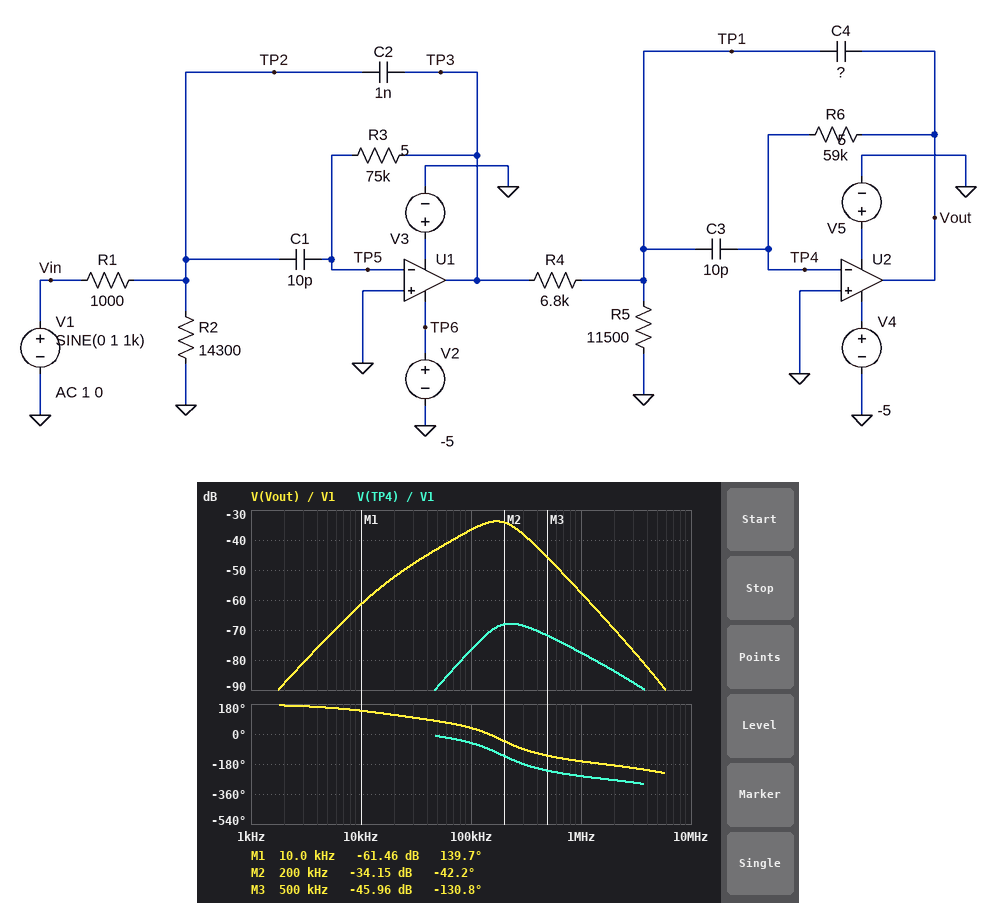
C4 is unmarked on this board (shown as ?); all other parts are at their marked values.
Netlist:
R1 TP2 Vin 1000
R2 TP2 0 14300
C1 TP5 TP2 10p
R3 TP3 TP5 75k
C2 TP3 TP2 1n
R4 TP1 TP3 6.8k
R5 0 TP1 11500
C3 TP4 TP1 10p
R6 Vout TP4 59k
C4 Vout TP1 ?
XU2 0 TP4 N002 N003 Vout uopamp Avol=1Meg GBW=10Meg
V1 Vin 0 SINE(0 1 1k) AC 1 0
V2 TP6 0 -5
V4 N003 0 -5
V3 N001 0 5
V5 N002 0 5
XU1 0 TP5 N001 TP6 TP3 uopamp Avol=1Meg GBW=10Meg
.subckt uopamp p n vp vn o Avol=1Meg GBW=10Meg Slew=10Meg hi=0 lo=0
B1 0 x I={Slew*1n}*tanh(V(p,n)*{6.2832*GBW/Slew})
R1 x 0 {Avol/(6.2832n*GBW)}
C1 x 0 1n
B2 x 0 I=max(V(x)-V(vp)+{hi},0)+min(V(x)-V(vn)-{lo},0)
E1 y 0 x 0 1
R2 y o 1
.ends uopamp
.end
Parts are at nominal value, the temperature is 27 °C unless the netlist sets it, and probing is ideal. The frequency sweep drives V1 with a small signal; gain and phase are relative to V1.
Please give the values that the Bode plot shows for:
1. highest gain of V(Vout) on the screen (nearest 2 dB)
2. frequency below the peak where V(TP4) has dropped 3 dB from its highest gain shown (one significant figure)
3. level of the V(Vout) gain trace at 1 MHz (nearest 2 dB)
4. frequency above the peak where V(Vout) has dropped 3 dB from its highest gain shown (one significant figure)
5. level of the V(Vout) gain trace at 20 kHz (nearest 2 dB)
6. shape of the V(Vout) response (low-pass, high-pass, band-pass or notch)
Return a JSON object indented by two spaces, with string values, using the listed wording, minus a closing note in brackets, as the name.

{
  "highest gain of V(Vout) on the screen": "-34 dB",
  "frequency below the peak where V(TP4) has dropped 3 dB from its highest gain shown": "100 kHz",
  "level of the V(Vout) gain trace at 1 MHz": "-58 dB",
  "frequency above the peak where V(Vout) has dropped 3 dB from its highest gain shown": "300 kHz",
  "level of the V(Vout) gain trace at 20 kHz": "-52 dB",
  "shape of the V(Vout) response": "band-pass"
}
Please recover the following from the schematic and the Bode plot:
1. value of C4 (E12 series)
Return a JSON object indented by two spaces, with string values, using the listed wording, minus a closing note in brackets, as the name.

{
  "value of C4": "2.7 nF"
}
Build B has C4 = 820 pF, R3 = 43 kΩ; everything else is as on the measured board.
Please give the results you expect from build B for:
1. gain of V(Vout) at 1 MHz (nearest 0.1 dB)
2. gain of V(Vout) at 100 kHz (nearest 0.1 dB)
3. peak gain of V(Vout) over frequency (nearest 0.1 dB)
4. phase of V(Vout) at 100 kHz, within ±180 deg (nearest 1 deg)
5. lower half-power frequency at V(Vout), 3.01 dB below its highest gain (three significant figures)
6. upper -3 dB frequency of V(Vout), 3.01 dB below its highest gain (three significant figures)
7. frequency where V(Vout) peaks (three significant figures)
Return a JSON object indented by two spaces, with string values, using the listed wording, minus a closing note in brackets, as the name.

{
  "gain of V(Vout) at 1 MHz": "-47.4 dB",
  "gain of V(Vout) at 100 kHz": "-31.8 dB",
  "peak gain of V(Vout) over frequency": "-28.4 dB",
  "phase of V(Vout) at 100 kHz, within ±180 deg": "58 deg",
  "lower half-power frequency at V(Vout), 3.01 dB below its highest gain": "105 kHz",
  "upper -3 dB frequency of V(Vout), 3.01 dB below its highest gain": "344 kHz",
  "frequency where V(Vout) peaks": "199 kHz"
}
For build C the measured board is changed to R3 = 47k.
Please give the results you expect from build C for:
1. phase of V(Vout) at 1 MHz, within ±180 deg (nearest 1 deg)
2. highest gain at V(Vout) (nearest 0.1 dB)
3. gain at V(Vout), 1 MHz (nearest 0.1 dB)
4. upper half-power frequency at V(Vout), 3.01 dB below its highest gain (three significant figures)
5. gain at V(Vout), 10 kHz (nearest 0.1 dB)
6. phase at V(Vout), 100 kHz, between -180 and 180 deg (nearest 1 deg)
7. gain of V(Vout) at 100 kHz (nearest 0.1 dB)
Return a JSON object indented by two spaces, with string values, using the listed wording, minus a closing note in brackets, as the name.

{
  "phase of V(Vout) at 1 MHz, within ±180 deg": "-157 deg",
  "highest gain at V(Vout)": "-38.4 dB",
  "gain at V(Vout), 1 MHz": "-57.7 dB",
  "upper half-power frequency at V(Vout), 3.01 dB below its highest gain": "337 kHz",
  "gain at V(Vout), 10 kHz": "-65.5 dB",
  "phase at V(Vout), 100 kHz, between -180 and 180 deg": "40 deg",
  "gain of V(Vout) at 100 kHz": "-41.4 dB"
}
